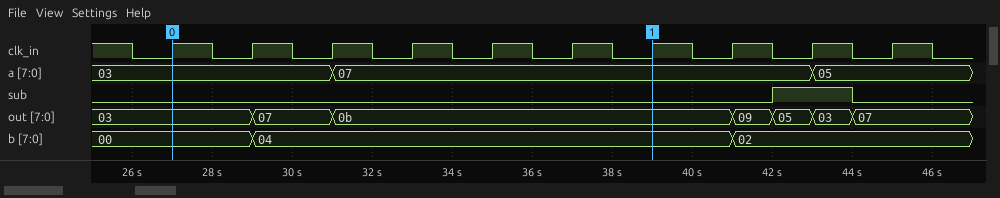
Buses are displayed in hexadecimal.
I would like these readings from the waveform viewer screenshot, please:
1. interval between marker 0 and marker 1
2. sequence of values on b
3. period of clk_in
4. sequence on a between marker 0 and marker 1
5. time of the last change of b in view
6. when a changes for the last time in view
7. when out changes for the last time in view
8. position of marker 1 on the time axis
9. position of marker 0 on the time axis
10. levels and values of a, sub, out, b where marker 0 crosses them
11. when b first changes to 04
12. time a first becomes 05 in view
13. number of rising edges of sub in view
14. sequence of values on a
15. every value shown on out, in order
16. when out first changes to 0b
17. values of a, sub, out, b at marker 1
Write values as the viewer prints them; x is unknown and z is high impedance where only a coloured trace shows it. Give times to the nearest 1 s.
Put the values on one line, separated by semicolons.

12 s; 00, 04, 02; 2 s; 03, 07; 41 s; 43 s; 44 s; 39 s; 27 s; a=03, sub=0, out=03, b=00; 29 s; 43 s; 1; 03, 07, 05; 03, 07, 0b, 09, 05, 03, 07; 31 s; a=07, sub=0, out=0b, b=04
